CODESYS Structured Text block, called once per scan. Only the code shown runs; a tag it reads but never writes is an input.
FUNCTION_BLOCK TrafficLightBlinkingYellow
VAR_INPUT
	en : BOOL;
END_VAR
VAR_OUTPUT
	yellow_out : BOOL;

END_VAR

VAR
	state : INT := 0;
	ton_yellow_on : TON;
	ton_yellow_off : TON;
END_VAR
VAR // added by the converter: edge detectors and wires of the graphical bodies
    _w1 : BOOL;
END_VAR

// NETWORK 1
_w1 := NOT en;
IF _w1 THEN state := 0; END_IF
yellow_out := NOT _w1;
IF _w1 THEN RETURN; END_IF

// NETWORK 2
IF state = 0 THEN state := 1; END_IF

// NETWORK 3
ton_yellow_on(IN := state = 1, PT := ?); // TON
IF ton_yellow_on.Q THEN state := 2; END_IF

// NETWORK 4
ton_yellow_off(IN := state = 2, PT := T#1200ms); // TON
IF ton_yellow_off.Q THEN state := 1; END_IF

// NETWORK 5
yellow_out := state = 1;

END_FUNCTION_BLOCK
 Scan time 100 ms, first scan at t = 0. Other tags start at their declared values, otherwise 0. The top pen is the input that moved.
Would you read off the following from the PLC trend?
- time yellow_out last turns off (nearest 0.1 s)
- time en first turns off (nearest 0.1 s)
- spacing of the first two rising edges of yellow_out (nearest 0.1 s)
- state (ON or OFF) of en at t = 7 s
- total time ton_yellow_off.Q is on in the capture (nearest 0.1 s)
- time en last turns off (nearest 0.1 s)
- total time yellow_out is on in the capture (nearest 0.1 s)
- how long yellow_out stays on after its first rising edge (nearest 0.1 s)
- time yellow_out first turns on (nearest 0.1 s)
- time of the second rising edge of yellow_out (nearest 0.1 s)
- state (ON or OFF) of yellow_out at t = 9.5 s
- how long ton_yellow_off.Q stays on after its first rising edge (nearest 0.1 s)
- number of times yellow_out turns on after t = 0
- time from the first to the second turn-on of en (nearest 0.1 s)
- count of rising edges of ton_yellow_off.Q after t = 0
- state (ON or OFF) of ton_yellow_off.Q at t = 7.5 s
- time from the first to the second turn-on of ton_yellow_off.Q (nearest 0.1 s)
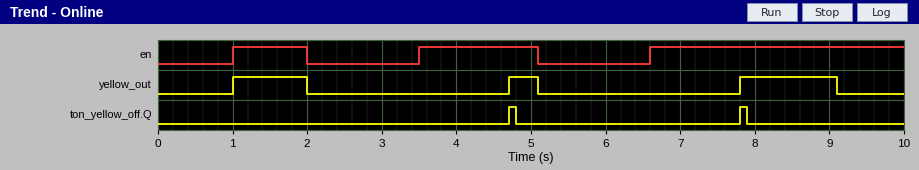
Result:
9.1 s
2.0 s
3.7 s
ON
0.2 s
5.1 s
2.7 s
1.0 s
1.0 s
4.7 s
OFF
0.1 s
3
2.5 s
2
OFF
3.1 s
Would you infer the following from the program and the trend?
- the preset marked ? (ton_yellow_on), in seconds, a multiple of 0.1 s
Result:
1.2 s
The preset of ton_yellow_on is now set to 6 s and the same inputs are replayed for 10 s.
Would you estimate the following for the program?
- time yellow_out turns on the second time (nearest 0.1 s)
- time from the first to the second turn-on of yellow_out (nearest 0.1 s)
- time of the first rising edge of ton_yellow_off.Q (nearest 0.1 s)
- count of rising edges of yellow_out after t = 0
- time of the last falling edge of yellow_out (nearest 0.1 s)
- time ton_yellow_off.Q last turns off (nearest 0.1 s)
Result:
3.5 s
2.5 s
8.2 s
4
7.0 s
8.3 s
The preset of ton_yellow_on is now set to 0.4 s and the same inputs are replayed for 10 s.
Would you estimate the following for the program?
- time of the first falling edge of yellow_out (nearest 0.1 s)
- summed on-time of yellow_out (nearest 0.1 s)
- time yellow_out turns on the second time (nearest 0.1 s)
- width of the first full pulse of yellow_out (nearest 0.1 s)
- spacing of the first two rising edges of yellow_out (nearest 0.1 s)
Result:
1.4 s
1.8 s
3.5 s
0.4 s
2.5 s
